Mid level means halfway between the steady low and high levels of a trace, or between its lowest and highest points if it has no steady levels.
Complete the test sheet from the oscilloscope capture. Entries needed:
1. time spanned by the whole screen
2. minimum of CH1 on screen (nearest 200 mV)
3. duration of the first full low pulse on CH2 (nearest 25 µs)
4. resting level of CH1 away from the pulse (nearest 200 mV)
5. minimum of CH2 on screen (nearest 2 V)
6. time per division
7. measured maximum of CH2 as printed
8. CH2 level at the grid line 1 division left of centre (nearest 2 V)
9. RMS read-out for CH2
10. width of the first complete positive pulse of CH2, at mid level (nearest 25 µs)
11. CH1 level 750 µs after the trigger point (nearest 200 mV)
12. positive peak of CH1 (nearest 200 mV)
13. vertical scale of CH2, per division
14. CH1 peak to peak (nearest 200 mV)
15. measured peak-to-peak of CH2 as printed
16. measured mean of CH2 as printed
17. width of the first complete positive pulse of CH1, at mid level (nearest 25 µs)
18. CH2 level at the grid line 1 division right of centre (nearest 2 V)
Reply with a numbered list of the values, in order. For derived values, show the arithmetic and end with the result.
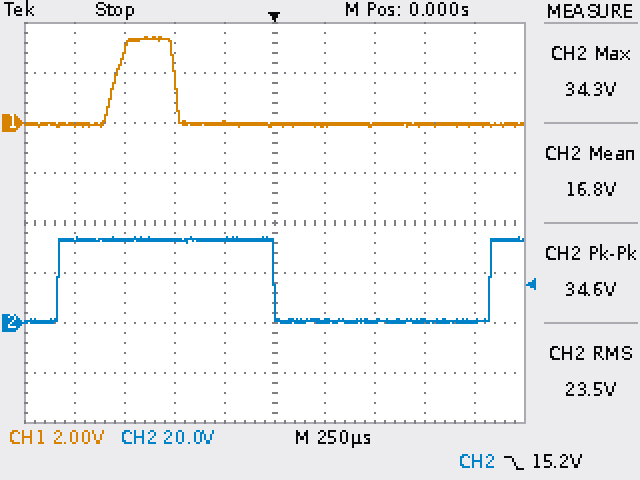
1. 2.5 ms
2. -200 mV
3. 1.075 ms
4. 0.0 V
5. 0 V
6. 250 µs
7. 34.3 V
8. 34 V
9. 23.5 V
10. 1.075 ms
11. 0.0 V
12. 3.4 V
13. 20 V
14. 3.4 V − (-200 mV) = 3.6 V
15. 34.6 V
16. 16.8 V
17. 300 µs
18. 0 V
